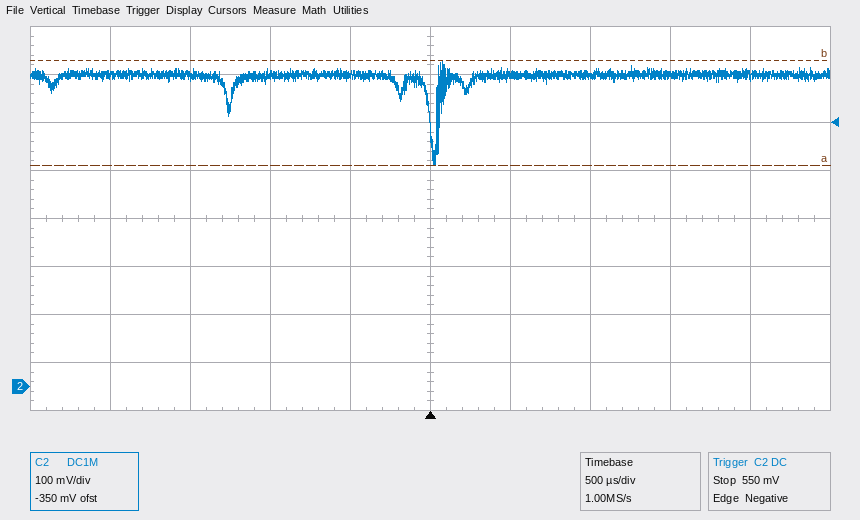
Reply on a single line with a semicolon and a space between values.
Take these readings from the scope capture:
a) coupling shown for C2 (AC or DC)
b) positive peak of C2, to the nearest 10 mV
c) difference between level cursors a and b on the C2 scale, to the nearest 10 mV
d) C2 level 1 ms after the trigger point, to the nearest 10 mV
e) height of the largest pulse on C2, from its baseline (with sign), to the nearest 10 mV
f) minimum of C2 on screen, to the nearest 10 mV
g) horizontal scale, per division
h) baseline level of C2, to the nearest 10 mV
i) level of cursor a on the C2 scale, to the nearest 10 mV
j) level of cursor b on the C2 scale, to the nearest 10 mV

DC; 680 mV; 220 mV; 650 mV; -190 mV; 460 mV; 500 µs; 650 mV; 460 mV; 680 mV
